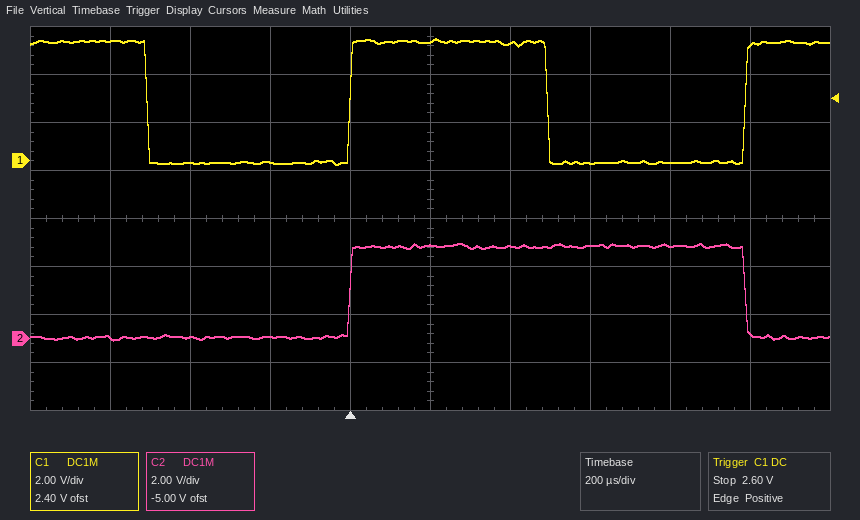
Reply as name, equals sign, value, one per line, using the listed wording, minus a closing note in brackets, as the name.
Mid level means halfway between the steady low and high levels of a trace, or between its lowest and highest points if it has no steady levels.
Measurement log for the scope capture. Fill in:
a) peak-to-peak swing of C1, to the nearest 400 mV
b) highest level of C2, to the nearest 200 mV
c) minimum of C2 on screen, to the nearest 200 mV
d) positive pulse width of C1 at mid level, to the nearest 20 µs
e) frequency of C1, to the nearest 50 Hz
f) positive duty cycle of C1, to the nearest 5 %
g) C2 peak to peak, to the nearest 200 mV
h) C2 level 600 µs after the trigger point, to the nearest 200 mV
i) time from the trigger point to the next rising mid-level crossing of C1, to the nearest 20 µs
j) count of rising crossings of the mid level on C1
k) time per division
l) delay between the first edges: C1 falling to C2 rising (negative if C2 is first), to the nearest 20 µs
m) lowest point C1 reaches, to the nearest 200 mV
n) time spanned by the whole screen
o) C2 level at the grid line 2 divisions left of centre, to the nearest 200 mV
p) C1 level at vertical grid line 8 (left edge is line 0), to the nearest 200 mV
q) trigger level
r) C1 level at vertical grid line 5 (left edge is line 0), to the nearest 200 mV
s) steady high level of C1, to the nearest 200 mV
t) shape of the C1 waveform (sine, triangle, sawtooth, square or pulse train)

peak-to-peak swing of C1, to the nearest 400 mV = 5.2 V
highest level of C2, to the nearest 200 mV = 4.0 V
minimum of C2 on screen, to the nearest 200 mV = 0.0 V
positive pulse width of C1 at mid level, to the nearest 20 µs = 500 µs
frequency of C1, to the nearest 50 Hz = 1.00 kHz
positive duty cycle of C1, to the nearest 5 % = 50 %
C2 peak to peak, to the nearest 200 mV = 4.0 V
C2 level 600 µs after the trigger point, to the nearest 200 mV = 3.8 V
time from the trigger point to the next rising mid-level crossing of C1, to the nearest 20 µs = 980 µs
count of rising crossings of the mid level on C1 = 2
time per division = 200 µs
delay between the first edges: C1 falling to C2 rising (negative if C2 is first), to the nearest 20 µs = +500 µs
lowest point C1 reaches, to the nearest 200 mV = -200 mV
time spanned by the whole screen = 2 ms
C2 level at the grid line 2 divisions left of centre, to the nearest 200 mV = 0.0 V
C1 level at vertical grid line 8 (left edge is line 0), to the nearest 200 mV = 0.0 V
trigger level = 2.60 V
C1 level at vertical grid line 5 (left edge is line 0), to the nearest 200 mV = 5.0 V
steady high level of C1, to the nearest 200 mV = 5.0 V
shape of the C1 waveform = square
